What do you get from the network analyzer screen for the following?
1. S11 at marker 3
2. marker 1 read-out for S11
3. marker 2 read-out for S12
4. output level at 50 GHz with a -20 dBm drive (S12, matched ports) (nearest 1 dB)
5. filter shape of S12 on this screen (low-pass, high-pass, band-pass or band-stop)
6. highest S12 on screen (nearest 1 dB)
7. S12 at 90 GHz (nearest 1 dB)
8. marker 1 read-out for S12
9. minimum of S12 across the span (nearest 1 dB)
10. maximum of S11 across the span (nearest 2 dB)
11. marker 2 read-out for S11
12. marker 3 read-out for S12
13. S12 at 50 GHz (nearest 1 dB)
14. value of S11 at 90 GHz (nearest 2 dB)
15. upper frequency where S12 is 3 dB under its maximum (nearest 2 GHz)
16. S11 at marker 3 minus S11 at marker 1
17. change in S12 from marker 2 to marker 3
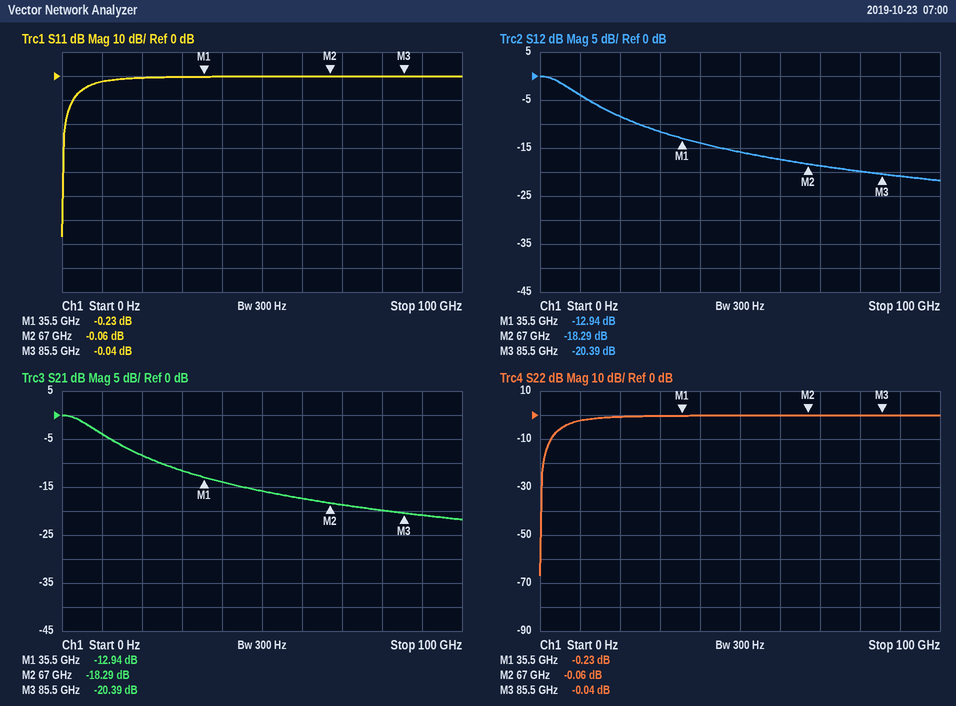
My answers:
-0.04 dB
-0.23 dB
-18.29 dB
-36 dBm
low-pass
0 dB
-21 dB
-12.94 dB
-22 dB
0 dB
-0.06 dB
-20.39 dB
-16 dB
0 dB
8 GHz
0.19 dB
-2.10 dB
